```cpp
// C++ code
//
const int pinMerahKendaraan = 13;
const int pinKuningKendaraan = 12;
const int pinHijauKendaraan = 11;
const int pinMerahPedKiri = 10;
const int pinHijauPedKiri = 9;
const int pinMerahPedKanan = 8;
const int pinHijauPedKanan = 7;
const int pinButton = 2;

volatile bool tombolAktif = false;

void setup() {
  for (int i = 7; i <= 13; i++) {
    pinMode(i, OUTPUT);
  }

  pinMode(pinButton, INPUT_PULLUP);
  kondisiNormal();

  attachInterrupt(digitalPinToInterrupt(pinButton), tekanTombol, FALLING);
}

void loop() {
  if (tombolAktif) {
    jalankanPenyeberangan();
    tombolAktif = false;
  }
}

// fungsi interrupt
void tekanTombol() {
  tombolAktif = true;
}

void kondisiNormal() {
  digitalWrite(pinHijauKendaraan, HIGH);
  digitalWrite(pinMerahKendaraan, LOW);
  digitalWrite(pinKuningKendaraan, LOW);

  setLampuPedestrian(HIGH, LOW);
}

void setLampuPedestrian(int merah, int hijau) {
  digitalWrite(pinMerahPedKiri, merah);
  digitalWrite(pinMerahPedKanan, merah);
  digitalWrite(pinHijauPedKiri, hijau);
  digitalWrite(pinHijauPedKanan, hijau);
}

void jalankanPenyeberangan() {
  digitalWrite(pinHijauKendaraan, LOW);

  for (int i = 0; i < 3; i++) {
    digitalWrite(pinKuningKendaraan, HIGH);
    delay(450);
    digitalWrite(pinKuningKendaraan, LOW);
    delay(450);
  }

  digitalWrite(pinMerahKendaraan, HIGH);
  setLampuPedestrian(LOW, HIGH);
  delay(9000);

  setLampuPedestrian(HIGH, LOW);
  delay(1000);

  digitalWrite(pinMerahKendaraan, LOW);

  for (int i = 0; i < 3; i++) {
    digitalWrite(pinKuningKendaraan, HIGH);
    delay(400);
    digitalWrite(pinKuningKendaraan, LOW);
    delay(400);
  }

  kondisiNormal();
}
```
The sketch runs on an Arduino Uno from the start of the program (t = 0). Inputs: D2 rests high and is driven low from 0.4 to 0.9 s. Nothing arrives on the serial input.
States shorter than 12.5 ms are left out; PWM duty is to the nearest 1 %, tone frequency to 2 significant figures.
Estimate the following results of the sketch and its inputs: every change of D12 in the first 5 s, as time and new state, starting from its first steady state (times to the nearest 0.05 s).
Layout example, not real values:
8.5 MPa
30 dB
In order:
0 s low; 0.4 s high; 0.85 s low; 1.3 s high; 1.75 s low; 2.2 s high; 2.65 s low
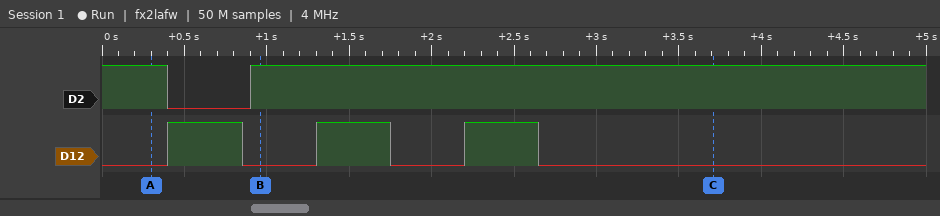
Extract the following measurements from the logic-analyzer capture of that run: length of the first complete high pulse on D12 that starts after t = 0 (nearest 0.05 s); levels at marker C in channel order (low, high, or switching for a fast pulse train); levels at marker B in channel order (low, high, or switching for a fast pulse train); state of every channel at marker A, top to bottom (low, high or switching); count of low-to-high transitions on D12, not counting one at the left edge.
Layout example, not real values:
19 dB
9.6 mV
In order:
0.45 s
D2 high, D12 low
D2 high, D12 low
D2 high, D12 low
3
